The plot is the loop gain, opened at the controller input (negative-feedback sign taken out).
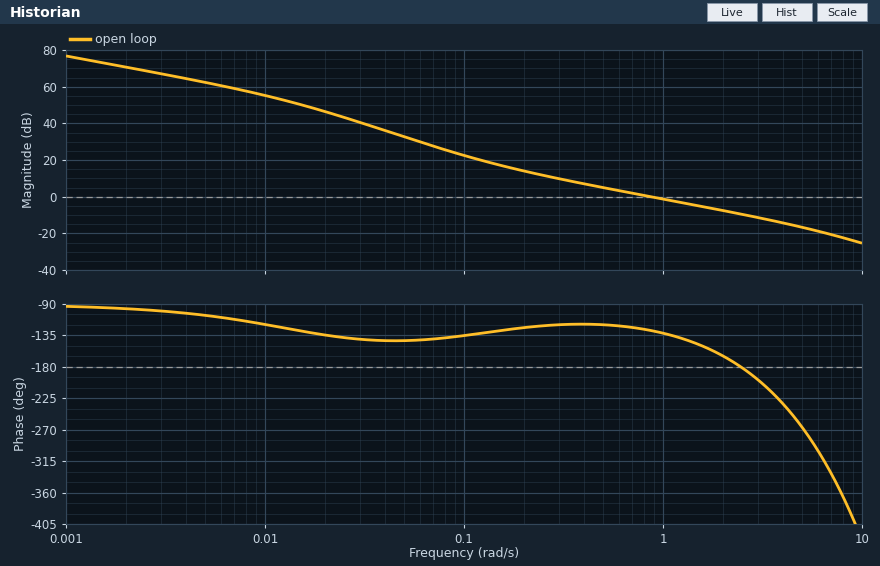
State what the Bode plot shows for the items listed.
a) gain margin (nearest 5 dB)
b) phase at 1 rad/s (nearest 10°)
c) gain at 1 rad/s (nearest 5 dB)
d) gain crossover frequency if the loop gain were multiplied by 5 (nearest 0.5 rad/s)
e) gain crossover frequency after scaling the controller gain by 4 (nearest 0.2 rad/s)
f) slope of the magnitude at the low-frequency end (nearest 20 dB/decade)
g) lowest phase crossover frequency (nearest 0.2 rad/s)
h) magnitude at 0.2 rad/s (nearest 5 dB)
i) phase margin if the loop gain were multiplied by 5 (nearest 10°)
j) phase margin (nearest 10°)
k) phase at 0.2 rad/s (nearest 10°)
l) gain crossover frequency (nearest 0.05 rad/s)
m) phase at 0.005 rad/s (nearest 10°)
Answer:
10 dB
-130°
0 dB
4.0 rad/s
3.2 rad/s
-20 dB/decade
2.4 rad/s
15 dB
-50°
50°
-120°
0.85 rad/s
-110°
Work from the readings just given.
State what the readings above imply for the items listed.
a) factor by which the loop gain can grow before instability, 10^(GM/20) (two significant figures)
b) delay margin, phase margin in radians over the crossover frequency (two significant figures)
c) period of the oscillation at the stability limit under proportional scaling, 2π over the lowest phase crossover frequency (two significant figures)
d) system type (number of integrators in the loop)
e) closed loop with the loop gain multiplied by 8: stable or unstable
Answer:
3.2
1.0 s
2.6 s
1
unstable
